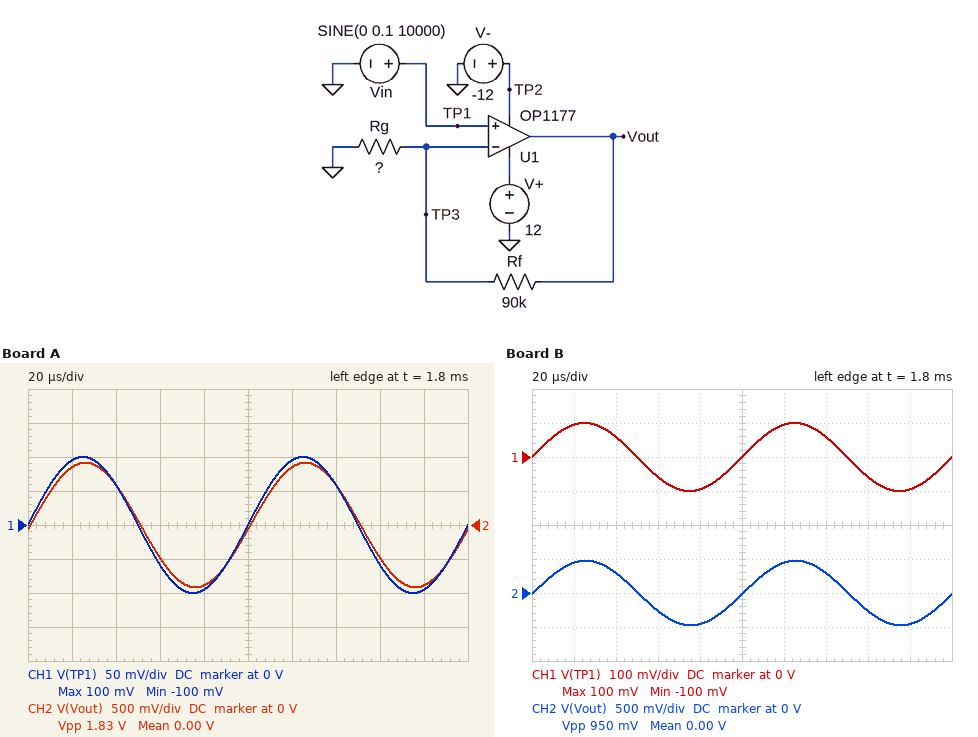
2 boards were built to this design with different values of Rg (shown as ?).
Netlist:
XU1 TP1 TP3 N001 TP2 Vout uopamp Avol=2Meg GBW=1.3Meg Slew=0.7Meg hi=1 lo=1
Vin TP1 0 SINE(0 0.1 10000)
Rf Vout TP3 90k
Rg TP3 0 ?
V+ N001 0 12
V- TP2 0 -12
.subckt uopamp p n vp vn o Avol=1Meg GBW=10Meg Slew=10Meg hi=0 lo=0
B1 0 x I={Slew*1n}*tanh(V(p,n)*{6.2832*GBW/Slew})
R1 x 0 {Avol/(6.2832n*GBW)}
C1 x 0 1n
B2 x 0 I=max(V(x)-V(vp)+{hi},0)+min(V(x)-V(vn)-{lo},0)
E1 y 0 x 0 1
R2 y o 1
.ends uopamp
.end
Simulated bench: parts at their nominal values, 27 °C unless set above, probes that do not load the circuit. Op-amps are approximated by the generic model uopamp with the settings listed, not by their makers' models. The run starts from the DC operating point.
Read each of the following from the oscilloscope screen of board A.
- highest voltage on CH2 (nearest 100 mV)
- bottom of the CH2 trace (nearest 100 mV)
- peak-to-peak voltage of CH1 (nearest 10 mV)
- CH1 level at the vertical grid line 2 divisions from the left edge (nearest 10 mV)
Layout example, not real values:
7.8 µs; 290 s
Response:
900 mV; -900 mV; 200 mV; 60 mV
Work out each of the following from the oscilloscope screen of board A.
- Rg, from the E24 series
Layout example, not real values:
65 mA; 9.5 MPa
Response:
11 kΩ
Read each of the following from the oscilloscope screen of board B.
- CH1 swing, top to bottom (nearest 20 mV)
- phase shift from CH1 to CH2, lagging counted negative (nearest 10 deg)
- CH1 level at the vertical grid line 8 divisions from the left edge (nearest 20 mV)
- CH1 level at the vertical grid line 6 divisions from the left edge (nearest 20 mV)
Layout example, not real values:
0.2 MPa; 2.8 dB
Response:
200 mV; 0 deg; -60 mV; 100 mV
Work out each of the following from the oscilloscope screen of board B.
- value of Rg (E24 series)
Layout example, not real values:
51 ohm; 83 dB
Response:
24 kΩ
